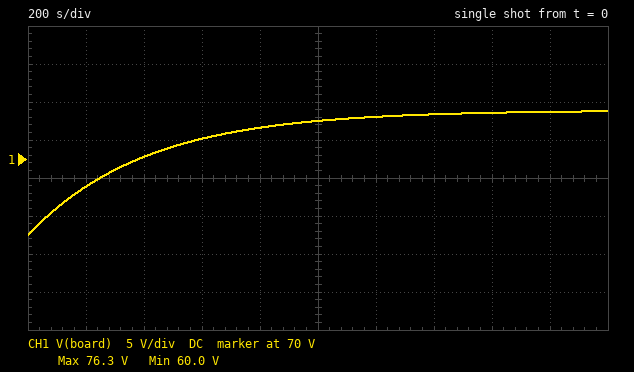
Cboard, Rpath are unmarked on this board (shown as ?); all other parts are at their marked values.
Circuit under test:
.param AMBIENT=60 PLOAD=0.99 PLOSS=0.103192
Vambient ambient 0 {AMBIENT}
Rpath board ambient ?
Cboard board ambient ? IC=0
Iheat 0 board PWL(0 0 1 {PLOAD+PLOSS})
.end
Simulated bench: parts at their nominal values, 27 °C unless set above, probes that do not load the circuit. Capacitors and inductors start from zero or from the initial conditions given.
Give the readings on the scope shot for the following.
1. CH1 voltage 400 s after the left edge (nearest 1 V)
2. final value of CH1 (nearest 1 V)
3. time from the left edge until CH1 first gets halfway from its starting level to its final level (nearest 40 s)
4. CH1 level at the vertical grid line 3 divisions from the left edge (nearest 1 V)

70 V
76 V
280 s
73 V
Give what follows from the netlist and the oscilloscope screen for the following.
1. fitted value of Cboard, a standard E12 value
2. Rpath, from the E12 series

27 F
15 Ω
